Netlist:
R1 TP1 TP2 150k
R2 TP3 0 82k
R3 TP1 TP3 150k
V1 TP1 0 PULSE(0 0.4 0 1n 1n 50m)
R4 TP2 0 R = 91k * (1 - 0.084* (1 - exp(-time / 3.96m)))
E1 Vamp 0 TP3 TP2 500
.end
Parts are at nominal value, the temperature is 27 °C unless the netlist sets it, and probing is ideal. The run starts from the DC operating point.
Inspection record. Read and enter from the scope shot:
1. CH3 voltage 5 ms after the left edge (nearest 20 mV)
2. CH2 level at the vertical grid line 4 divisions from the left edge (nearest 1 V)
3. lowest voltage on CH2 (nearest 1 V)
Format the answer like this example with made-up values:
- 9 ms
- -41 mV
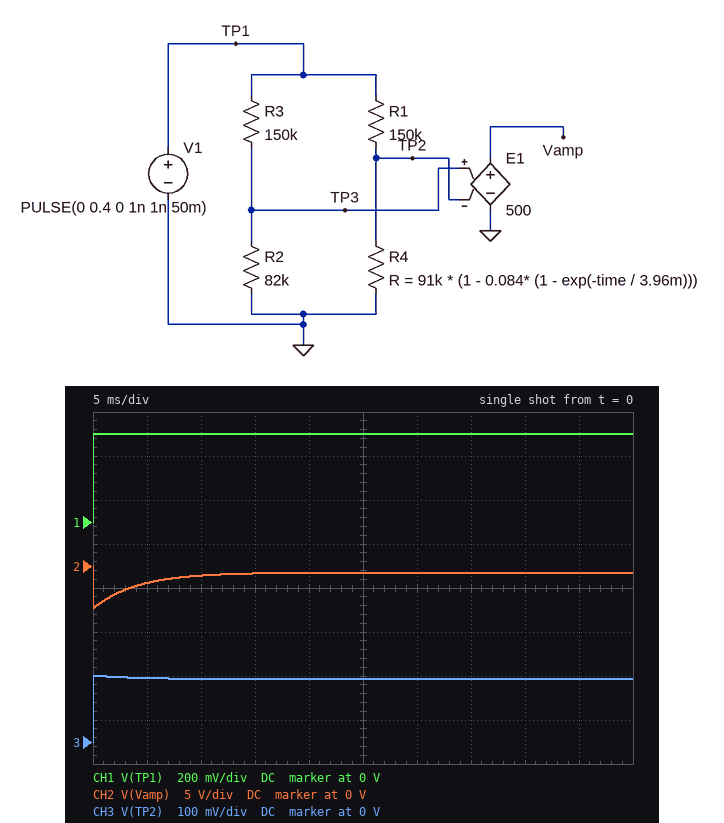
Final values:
- 140 mV
- -1 V
- -5 V
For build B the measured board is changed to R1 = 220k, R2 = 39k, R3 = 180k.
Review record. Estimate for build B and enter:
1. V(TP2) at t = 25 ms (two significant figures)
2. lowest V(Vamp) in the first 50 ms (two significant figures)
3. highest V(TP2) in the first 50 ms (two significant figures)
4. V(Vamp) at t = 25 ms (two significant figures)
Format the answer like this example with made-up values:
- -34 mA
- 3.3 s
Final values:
- 110 mV
- -23 V
- 120 mV
- -19 V
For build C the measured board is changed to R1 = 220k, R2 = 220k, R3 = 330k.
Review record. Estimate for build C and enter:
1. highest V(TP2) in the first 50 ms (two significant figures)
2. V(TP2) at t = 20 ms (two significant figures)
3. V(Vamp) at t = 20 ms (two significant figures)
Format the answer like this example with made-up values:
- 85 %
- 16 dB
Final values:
- 120 mV
- 110 mV
- 25 V
